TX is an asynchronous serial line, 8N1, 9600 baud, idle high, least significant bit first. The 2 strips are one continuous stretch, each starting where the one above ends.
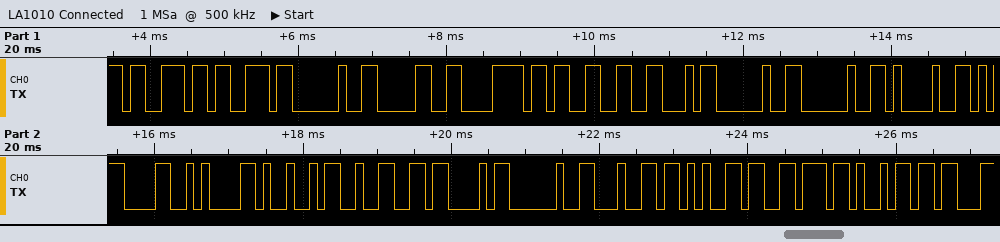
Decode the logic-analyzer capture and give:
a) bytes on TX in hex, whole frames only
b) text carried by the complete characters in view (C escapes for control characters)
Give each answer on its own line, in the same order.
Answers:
73 73 20 30 78 33 46 20 20 21 0D 0A 49 32 43 20 64 65 76 69
"ss 0x3F  !\r\nI2C devi"
